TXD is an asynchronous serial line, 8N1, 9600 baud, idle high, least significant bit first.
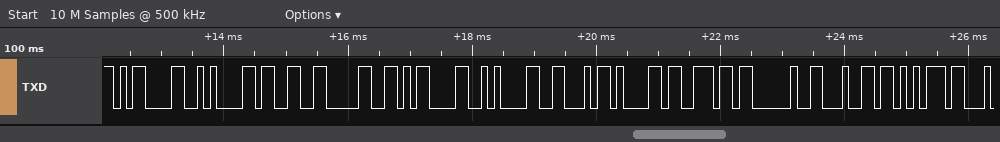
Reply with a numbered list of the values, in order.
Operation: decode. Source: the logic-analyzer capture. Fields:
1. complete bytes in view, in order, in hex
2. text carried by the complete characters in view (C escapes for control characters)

1. 0D 0A 33 30 0D 0A 46 61 6E 20 64 75
2. "\r\n30\r\nFan du"
